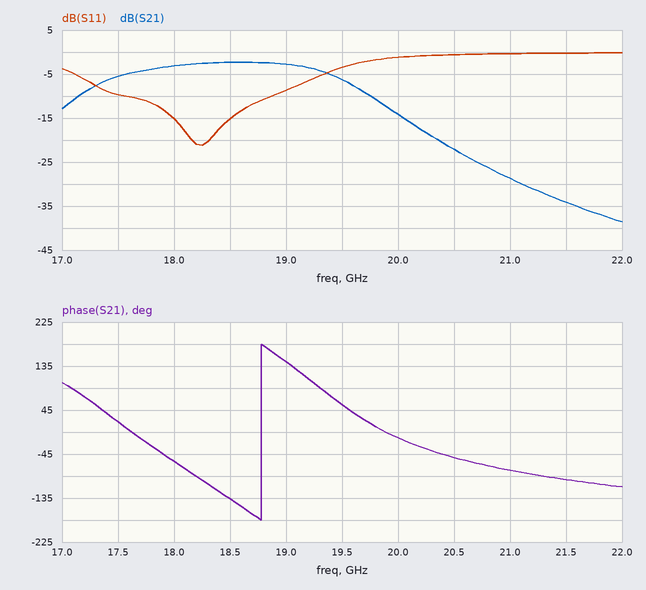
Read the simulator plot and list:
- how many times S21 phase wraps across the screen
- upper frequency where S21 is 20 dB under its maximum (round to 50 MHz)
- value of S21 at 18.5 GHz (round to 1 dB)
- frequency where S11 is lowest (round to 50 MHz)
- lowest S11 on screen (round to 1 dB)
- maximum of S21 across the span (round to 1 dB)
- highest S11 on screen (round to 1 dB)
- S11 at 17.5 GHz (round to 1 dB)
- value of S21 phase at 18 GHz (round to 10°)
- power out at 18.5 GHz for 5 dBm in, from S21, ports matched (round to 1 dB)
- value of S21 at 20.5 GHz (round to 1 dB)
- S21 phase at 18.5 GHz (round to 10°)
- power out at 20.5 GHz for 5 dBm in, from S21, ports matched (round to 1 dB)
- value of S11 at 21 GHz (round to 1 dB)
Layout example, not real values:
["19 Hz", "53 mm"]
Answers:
["1", "20.50 GHz", "-2 dB", "18.25 GHz", "-21 dB", "-2 dB", "0 dB", "-10 dB", "-60°", "3 dBm", "-22 dB", "-140°", "-17 dBm", "0 dB"]
